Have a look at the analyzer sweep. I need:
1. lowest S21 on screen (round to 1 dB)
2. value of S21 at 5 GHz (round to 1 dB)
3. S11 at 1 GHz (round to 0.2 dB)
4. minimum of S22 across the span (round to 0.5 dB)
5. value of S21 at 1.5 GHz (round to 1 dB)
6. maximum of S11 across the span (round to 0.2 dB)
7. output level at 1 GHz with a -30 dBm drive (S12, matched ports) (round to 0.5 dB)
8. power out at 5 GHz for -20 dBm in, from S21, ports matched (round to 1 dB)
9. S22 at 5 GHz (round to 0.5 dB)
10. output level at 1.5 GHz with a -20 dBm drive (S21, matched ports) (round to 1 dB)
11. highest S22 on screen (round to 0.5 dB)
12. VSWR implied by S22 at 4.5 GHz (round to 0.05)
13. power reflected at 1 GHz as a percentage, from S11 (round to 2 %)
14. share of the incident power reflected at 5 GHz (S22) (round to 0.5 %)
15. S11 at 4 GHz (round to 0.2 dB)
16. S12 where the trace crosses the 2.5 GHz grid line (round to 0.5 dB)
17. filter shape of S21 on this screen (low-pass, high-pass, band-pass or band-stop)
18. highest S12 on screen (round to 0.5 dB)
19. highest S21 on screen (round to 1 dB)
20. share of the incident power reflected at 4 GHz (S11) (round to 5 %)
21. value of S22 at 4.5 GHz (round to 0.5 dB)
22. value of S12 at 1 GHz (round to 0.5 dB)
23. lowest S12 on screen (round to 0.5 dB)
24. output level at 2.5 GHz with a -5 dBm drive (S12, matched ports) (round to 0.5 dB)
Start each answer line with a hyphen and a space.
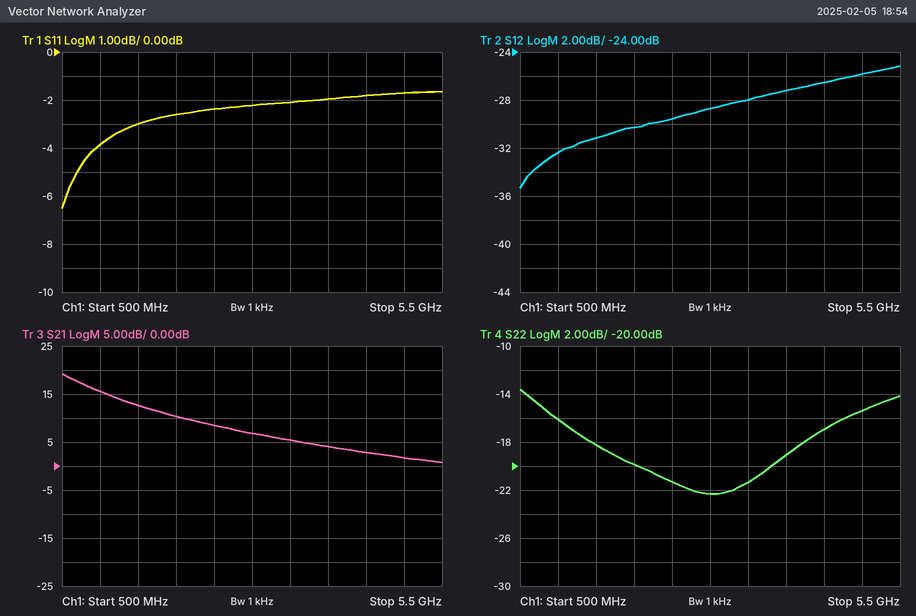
- 1 dB
- 2 dB
- -3.8 dB
- -22.5 dB
- 13 dB
- -1.6 dB
- -62.5 dBm
- -18 dBm
- -15.5 dB
- -7 dBm
- -13.5 dB
- 1.35
- 42 %
- 3.0 %
- -2.0 dB
- -29.5 dB
- low-pass
- -25.0 dB
- 19 dB
- 65 %
- -17.0 dB
- -32.5 dB
- -35.5 dB
- -34.5 dBm
